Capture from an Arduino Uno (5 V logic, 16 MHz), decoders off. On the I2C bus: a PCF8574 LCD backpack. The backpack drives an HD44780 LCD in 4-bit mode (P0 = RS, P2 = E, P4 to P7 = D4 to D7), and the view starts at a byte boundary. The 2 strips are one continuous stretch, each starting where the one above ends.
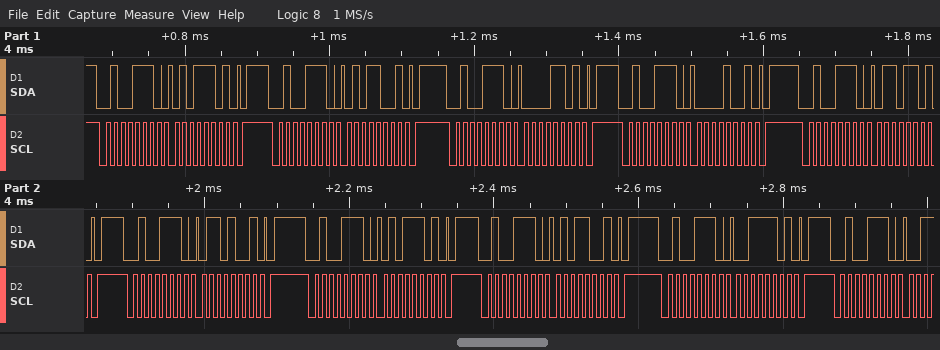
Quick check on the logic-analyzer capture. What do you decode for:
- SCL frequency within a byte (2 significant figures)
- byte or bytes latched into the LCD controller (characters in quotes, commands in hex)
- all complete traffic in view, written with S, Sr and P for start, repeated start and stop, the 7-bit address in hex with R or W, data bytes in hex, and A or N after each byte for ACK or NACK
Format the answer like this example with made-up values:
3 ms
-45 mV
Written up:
100 kHz
'P' 'e'
S 27W A 5D A P S 27W A 59 A P S 27W A 0D A P S 27W A 09 A P S 27W A 6D A P S 27W A 69 A P S 27W A 5D A P S 27W A 59 A P S 27W A 3D A P S 27W A
